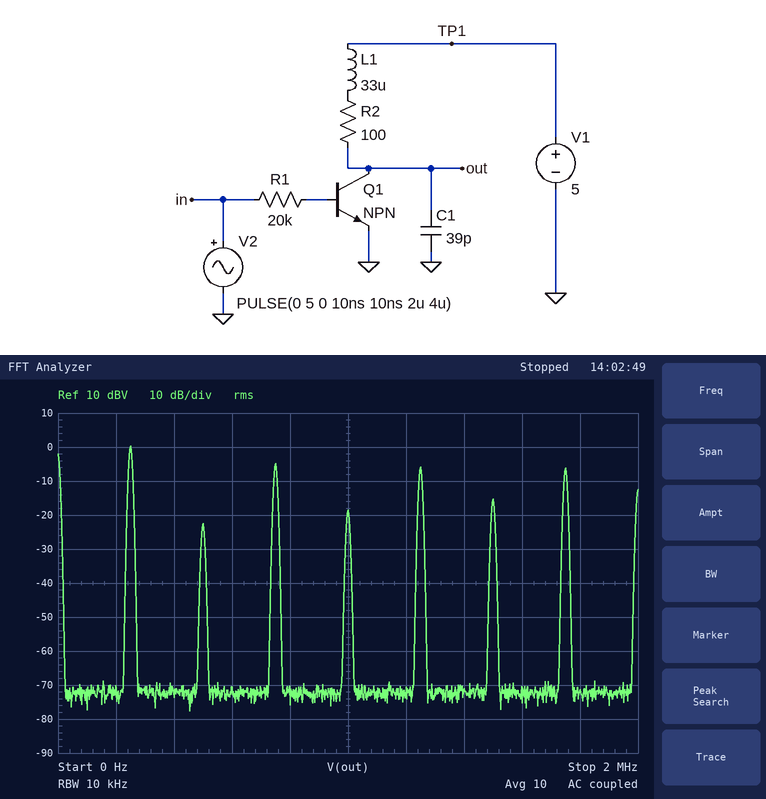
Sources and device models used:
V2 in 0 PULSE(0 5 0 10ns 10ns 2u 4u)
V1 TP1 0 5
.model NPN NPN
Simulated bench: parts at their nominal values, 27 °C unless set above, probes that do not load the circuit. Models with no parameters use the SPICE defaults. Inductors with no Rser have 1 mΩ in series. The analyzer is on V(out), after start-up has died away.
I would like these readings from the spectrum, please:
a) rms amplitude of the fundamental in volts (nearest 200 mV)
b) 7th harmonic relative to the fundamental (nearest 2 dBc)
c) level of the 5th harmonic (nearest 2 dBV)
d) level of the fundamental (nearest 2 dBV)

1.0 V
-6 dBc
-6 dBV
0 dBV
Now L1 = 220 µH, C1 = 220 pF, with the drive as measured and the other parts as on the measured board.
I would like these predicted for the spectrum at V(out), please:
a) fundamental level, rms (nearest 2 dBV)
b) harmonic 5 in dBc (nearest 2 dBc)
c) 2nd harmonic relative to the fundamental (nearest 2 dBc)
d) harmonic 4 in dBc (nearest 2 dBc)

10 dBV
-8 dBc
4 dBc
-2 dBc
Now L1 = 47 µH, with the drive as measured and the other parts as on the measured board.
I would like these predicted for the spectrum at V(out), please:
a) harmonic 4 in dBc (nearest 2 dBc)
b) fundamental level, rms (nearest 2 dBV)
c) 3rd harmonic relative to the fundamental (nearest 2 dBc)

-12 dBc
2 dBV
-4 dBc
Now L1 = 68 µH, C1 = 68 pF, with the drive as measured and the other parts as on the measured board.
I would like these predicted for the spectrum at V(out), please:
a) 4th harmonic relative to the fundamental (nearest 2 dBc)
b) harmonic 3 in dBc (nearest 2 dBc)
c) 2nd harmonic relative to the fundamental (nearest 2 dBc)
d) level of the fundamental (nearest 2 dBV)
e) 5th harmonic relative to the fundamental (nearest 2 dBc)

-6 dBc
-2 dBc
-12 dBc
2 dBV
-4 dBc
